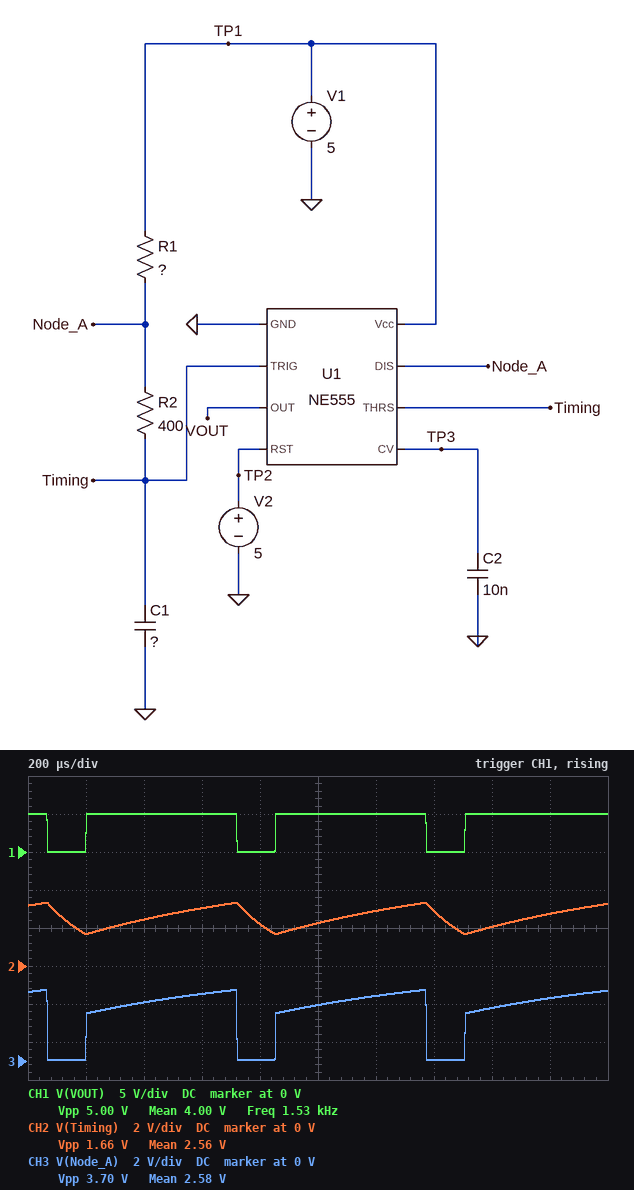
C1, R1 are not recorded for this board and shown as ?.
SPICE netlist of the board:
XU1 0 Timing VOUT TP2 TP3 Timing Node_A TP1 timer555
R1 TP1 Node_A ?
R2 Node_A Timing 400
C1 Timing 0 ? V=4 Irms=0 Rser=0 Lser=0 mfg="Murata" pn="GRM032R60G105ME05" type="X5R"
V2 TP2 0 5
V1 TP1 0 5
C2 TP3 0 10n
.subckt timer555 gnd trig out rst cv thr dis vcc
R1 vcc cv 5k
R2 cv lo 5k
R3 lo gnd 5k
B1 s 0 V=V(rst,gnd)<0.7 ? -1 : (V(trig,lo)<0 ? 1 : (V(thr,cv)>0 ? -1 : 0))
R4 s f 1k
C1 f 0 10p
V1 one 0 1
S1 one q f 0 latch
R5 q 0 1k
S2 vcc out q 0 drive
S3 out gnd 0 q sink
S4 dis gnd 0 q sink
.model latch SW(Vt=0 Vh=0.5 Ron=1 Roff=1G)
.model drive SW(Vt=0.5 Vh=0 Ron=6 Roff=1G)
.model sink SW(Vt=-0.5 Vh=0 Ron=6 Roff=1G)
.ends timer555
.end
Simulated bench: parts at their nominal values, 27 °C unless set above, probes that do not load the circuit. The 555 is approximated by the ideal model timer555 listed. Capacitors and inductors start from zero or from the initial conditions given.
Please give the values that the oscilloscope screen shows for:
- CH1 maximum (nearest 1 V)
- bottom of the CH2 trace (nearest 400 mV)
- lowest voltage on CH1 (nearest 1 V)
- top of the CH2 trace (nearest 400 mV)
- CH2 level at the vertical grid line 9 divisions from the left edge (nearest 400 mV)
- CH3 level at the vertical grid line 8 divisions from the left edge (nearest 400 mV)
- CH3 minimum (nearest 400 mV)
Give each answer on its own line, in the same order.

5 V
1.6 V
0 V
3.2 V
2.8 V
2.8 V
0 V
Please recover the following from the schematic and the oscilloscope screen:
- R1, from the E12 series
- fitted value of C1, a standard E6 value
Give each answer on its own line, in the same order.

1.2 kΩ
470 nF
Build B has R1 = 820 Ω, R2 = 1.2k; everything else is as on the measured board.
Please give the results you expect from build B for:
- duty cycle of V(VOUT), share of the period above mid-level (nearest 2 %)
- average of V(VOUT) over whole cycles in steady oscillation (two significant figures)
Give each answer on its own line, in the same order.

62 %
3.1 V
